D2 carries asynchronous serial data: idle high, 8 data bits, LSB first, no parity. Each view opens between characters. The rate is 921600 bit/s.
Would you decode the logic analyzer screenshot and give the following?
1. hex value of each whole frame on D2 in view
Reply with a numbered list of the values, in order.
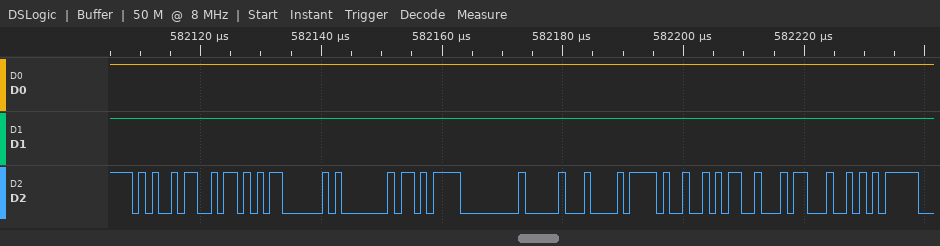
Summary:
1. A5, 5A, 03, 01, EB, 00, 10, E8, 49, 13, 23, F5
